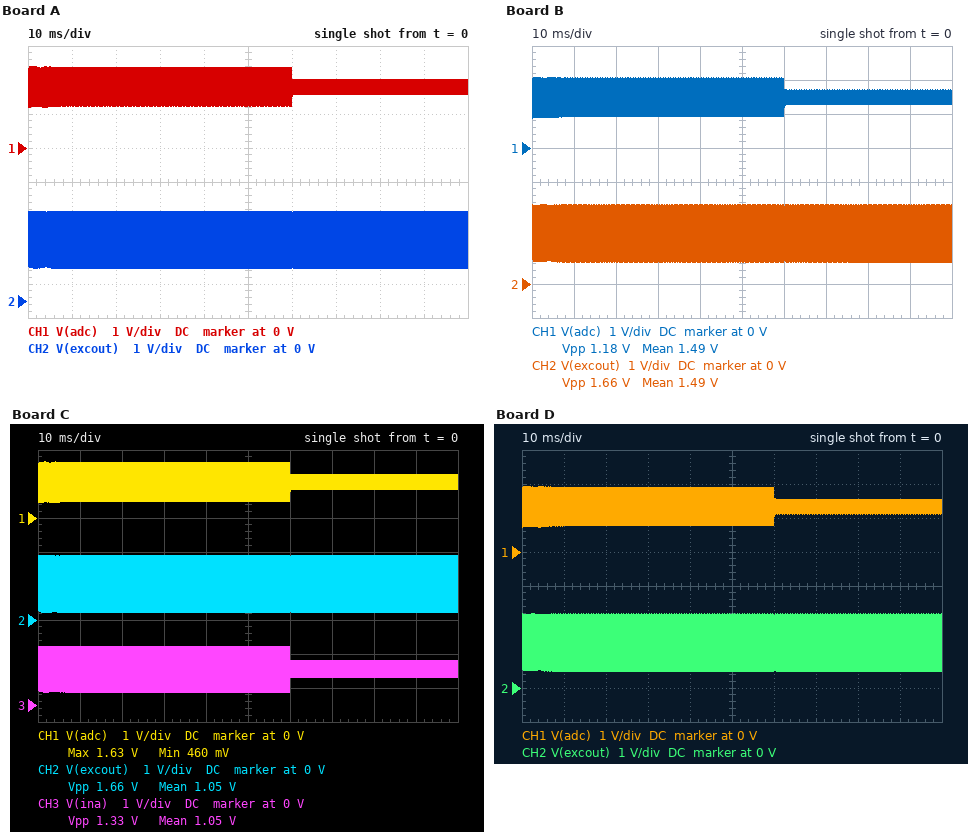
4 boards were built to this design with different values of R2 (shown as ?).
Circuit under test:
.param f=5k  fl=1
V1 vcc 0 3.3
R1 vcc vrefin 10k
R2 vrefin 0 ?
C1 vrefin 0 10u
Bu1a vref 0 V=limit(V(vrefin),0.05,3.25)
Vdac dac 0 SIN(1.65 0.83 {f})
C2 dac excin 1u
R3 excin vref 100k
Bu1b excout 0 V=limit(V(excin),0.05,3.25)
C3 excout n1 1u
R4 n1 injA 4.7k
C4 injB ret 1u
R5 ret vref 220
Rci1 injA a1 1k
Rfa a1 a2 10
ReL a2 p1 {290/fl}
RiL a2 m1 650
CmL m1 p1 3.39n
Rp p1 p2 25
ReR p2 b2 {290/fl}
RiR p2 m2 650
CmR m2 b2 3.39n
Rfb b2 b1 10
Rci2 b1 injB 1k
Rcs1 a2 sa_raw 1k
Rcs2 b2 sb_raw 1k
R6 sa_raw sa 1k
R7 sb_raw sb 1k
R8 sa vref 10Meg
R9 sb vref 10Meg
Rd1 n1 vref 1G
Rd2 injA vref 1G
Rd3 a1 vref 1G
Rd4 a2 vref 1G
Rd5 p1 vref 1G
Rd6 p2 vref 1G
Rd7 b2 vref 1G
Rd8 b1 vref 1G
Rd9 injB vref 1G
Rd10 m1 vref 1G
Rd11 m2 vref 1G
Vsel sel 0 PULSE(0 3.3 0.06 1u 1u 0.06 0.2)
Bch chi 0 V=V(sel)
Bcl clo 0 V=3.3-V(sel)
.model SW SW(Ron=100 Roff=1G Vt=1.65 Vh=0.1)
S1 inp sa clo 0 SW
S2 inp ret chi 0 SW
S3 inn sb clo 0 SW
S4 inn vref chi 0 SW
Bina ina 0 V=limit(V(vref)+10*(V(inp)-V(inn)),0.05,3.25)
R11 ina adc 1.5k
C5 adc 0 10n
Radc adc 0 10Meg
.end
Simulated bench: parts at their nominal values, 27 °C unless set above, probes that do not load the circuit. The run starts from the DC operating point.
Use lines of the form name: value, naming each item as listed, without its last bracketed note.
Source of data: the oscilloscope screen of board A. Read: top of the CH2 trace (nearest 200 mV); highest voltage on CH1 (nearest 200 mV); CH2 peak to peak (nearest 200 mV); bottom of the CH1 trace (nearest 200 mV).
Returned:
top of the CH2 trace: 2.6 V
highest voltage on CH1: 2.4 V
CH2 peak to peak: 1.6 V
bottom of the CH1 trace: 1.2 V
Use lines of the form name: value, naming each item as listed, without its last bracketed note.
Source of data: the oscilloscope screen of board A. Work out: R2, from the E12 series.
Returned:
R2, from the E12 series: 12 kΩ
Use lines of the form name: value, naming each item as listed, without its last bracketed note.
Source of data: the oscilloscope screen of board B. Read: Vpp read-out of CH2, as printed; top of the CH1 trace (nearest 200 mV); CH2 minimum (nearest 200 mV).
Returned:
Vpp read-out of CH2, as printed: 1.66 V
top of the CH1 trace: 2.0 V
CH2 minimum: 600 mV
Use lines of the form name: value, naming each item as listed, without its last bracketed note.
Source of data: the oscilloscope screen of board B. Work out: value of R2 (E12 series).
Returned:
value of R2: 8.2 kΩ
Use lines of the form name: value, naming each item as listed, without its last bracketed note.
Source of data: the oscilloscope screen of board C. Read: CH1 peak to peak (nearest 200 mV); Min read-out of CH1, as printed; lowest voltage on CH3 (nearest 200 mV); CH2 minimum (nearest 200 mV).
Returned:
CH1 peak to peak: 1.2 V
Min read-out of CH1, as printed: 460 mV
lowest voltage on CH3: 400 mV
CH2 minimum: 200 mV
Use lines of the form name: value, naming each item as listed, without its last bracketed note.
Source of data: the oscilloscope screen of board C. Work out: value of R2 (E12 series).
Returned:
value of R2: 4.7 kΩ
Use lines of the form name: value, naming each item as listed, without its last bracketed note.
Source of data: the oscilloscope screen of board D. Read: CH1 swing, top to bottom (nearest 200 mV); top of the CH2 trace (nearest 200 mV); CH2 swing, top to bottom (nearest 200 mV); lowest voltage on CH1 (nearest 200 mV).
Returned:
CH1 swing, top to bottom: 1.2 V
top of the CH2 trace: 2.2 V
CH2 swing, top to bottom: 1.6 V
lowest voltage on CH1: 800 mV
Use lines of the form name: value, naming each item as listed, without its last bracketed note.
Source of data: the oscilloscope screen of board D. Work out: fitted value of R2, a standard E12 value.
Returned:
fitted value of R2, a standard E12 value: 6.8 kΩ
